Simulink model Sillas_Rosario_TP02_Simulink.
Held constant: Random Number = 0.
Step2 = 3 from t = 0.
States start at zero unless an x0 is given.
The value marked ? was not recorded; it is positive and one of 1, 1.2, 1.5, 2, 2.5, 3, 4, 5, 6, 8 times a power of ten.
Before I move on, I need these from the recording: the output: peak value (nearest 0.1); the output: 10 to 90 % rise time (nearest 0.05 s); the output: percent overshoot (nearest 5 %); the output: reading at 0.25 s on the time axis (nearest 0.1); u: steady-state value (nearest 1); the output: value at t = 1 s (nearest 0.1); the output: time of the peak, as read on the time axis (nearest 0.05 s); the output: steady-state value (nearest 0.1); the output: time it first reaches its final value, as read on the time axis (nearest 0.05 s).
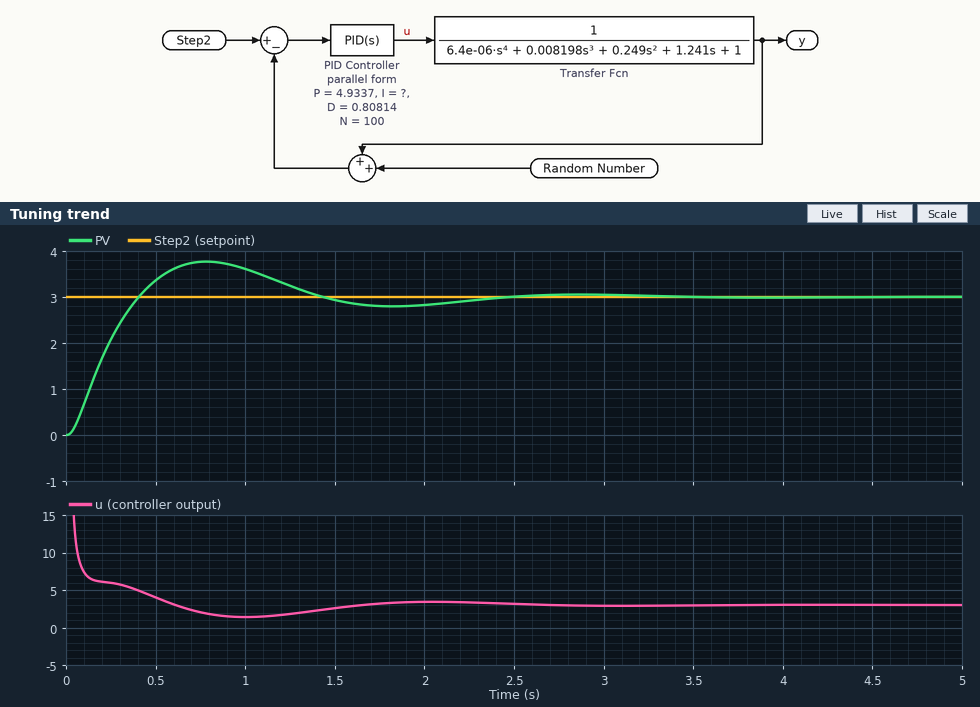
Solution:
3.8
0.30 s
25 %
2.1
3
3.6
0.80 s
3.0
0.40 s
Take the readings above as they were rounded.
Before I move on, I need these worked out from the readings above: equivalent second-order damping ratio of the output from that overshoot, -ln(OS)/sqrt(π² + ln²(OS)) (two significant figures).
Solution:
0.40
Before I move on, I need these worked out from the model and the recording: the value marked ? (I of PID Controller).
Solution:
15
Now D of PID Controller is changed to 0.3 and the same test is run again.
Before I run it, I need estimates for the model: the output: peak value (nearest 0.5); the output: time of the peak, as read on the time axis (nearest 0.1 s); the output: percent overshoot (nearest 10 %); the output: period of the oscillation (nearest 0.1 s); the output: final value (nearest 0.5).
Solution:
4.5
0.7 s
50 %
1.6 s
3.0
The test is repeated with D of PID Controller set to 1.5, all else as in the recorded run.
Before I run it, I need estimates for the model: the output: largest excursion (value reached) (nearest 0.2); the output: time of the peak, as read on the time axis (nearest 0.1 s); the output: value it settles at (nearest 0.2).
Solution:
3.4
1.0 s
3.0
